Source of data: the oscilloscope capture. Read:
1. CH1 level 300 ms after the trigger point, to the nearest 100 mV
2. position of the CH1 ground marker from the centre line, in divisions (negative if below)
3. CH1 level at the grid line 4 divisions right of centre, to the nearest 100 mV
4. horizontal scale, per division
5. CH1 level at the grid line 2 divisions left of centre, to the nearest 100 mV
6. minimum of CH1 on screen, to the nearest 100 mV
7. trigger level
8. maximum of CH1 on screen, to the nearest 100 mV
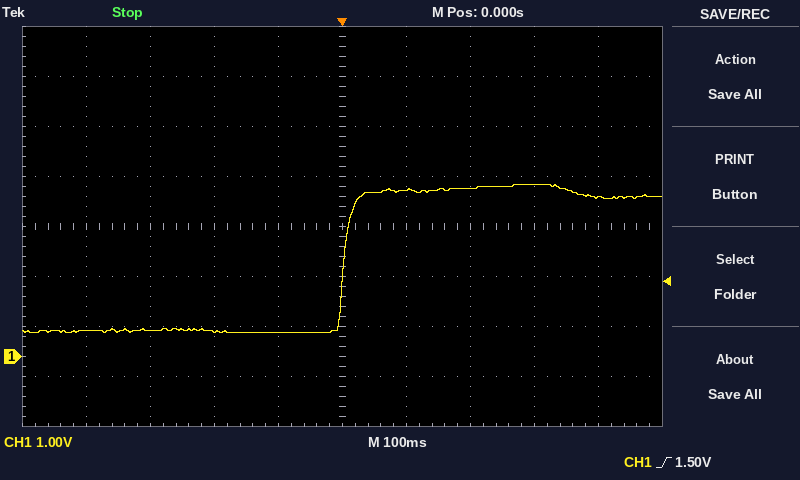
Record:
3.4 V
-2.6 div
3.2 V
100 ms
500 mV
500 mV
1.50 V
3.4 V
